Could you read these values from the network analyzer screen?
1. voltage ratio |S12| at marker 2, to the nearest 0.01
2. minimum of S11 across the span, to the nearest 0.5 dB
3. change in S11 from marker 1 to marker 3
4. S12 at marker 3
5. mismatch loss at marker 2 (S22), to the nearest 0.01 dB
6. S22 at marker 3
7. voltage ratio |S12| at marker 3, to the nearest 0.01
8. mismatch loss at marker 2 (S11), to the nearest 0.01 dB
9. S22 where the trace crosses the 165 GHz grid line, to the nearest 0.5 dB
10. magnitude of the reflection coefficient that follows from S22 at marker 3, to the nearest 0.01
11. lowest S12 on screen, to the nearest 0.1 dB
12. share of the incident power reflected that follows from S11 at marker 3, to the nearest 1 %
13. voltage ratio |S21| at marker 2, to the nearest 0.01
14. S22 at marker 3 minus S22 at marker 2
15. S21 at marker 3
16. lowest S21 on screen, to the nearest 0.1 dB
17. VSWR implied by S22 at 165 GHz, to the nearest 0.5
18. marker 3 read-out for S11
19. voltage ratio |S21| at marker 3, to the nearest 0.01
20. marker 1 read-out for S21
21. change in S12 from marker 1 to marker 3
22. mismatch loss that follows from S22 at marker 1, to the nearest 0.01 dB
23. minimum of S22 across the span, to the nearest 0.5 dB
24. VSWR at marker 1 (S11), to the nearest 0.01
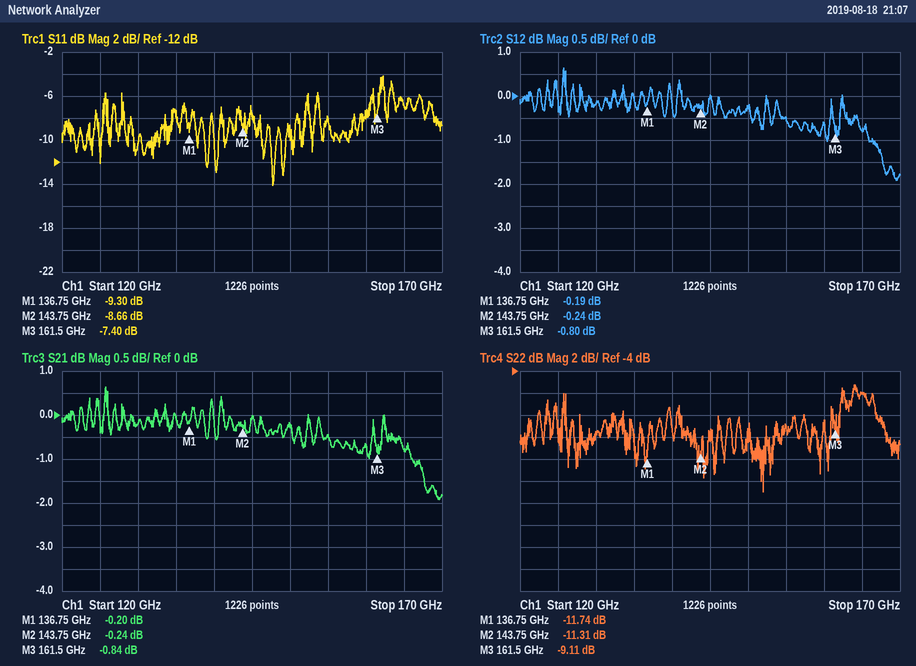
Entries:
0.97
-14.0 dB
1.90 dB
-0.80 dB
0.33 dB
-9.11 dB
0.91
0.64 dB
-6.0 dB
0.35
-1.9 dB
18 %
0.97
2.20 dB
-0.84 dB
-1.9 dB
3.0
-7.40 dB
0.91
-0.20 dB
-0.61 dB
0.30 dB
-15.0 dB
2.04
